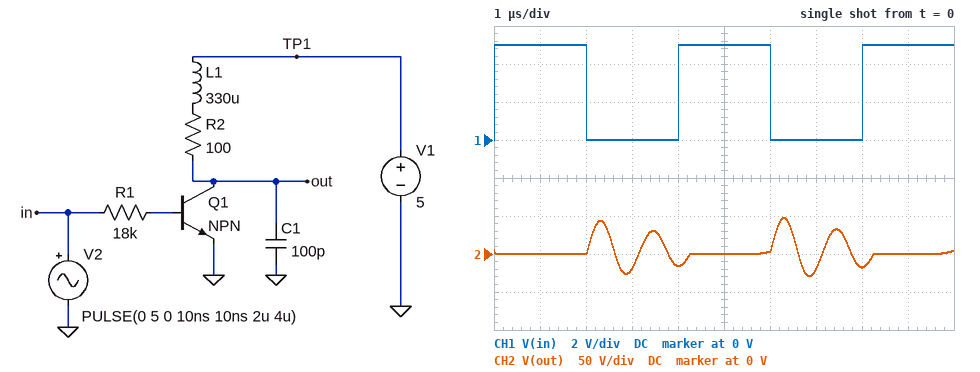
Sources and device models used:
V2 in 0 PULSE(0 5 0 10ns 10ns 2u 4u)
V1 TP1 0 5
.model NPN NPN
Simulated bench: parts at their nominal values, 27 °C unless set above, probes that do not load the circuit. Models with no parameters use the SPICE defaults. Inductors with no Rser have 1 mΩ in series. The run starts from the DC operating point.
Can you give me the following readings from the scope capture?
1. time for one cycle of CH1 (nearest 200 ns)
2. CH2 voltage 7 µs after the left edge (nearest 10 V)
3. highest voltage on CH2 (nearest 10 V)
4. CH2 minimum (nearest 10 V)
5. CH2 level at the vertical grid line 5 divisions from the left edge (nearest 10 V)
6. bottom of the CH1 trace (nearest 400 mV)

4.0 µs
-20 V
50 V
-30 V
0 V
0 V
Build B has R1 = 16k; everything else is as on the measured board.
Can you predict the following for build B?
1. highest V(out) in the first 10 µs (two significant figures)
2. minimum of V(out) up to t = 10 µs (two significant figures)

49 V
-30 V
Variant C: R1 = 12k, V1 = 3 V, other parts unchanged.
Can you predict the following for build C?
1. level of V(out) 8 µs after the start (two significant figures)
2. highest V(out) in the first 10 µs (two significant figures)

-8.8 V
28 V
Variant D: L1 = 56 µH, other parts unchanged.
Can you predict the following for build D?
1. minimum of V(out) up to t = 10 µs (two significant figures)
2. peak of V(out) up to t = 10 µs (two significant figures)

-7.3 V
21 V
